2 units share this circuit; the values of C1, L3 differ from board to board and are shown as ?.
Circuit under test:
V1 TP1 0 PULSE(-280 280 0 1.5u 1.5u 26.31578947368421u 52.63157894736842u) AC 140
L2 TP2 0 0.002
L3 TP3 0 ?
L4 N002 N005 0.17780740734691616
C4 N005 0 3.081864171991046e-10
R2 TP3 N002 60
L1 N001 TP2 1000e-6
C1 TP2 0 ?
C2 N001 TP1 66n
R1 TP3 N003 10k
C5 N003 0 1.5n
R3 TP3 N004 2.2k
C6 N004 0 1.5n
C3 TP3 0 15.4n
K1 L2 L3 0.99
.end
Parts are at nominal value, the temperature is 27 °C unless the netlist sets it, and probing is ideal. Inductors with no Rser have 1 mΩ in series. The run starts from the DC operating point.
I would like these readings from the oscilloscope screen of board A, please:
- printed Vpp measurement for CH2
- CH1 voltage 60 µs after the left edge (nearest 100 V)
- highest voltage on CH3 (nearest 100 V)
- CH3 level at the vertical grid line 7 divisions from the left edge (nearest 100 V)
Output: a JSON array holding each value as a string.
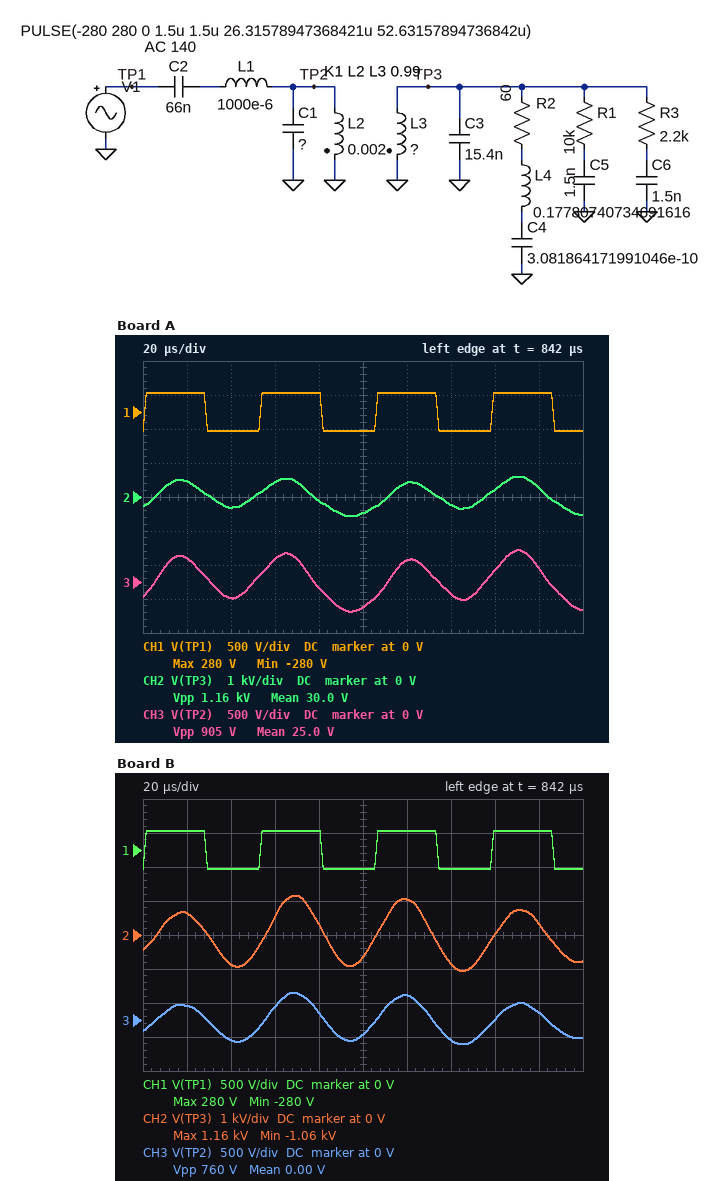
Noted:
["1.16 kV", "300 V", "500 V", "-200 V"]
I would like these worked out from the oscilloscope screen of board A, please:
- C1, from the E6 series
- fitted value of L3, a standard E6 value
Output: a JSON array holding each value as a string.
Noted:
["47 nF", "3.3 mH"]
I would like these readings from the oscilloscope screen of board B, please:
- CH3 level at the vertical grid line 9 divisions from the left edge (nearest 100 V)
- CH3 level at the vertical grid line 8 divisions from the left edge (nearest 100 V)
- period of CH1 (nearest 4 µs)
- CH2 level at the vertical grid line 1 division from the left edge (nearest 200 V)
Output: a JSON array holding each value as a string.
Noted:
["100 V", "0 V", "52 µs", "600 V"]
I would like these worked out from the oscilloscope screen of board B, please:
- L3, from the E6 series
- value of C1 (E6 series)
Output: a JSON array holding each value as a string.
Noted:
["15 mH", "100 nF"]
